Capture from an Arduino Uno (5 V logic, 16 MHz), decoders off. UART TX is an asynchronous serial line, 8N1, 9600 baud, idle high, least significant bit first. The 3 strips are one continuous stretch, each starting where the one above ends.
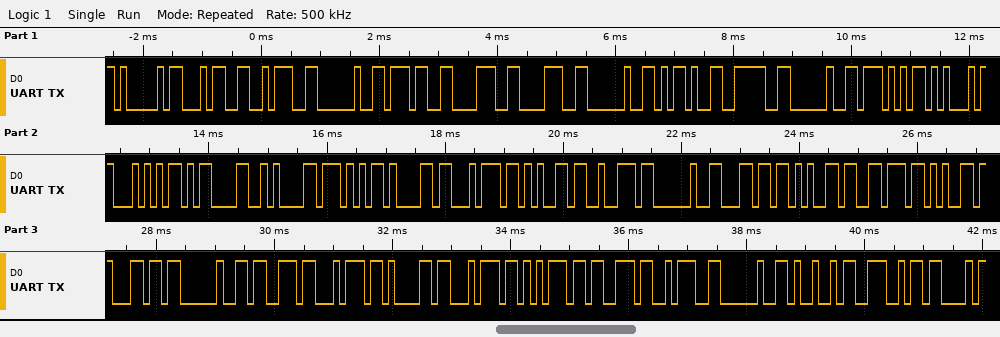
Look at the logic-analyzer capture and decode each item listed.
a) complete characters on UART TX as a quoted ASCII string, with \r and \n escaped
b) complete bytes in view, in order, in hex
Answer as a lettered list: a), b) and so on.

a) "A4: 788 -> WET\r\nWater level status: INC"
b) 0x41 0x34 0x3A 0x20 0x37 0x38 0x38 0x20 0x2D 0x3E 0x20 0x57 0x45 0x54 0x0D 0x0A 0x57 0x61 0x74 0x65 0x72 0x20 0x6C 0x65 0x76 0x65 0x6C 0x20 0x73 0x74 0x61 0x74 0x75 0x73 0x3A 0x20 0x49 0x4E 0x43
